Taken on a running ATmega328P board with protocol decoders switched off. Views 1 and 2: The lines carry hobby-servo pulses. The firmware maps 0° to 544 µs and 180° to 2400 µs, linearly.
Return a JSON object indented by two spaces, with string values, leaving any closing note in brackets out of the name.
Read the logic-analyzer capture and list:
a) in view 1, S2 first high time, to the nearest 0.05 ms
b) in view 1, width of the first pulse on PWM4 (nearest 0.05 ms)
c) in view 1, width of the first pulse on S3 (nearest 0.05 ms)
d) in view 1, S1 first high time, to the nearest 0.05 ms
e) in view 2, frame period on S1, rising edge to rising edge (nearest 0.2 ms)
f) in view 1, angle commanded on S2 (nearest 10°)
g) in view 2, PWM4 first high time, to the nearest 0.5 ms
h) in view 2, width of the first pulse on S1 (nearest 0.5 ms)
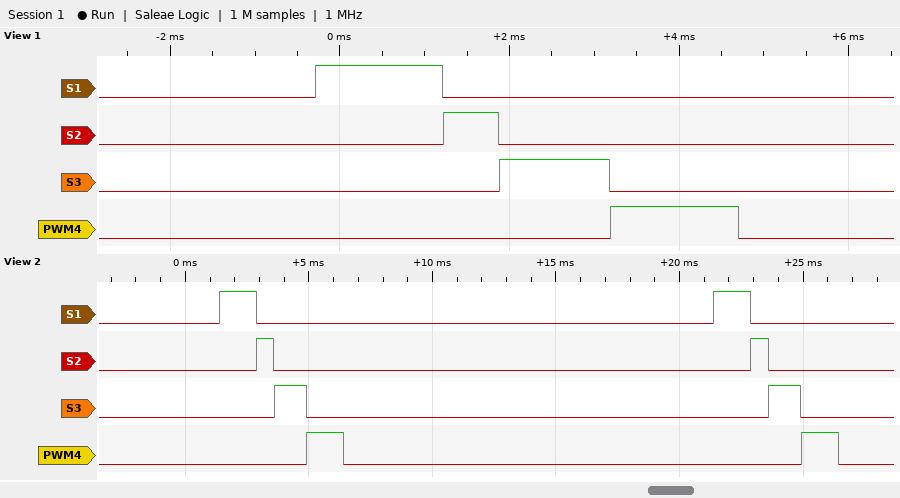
{
  "in view 1, S2 first high time, to the nearest 0.05 ms": "0.65 ms",
  "in view 1, width of the first pulse on PWM4": "1.50 ms",
  "in view 1, width of the first pulse on S3": "1.30 ms",
  "in view 1, S1 first high time, to the nearest 0.05 ms": "1.50 ms",
  "in view 2, frame period on S1, rising edge to rising edge": "20.0 ms",
  "in view 1, angle commanded on S2": "10°",
  "in view 2, PWM4 first high time, to the nearest 0.5 ms": "1.5 ms",
  "in view 2, width of the first pulse on S1": "1.5 ms"
}
